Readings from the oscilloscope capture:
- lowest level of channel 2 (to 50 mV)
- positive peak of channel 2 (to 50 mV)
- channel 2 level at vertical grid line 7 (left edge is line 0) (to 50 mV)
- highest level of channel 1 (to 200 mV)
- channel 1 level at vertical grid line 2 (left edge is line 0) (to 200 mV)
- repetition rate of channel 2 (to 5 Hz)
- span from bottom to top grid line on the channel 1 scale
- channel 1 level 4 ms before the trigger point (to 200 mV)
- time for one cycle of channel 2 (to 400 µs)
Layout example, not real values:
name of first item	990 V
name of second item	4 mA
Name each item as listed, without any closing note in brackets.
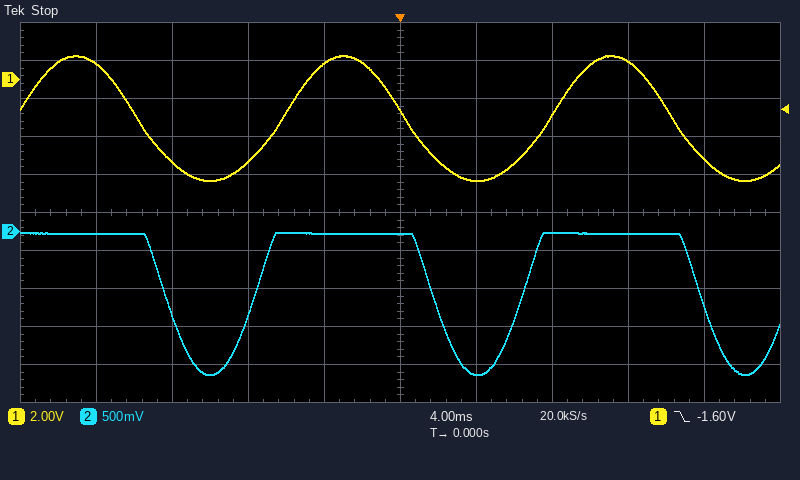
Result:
lowest level of channel 2	-1.90 V
positive peak of channel 2	0 mV
channel 2 level at vertical grid line 7 (left edge is line 0)	0 mV
highest level of channel 1	1.2 V
channel 1 level at vertical grid line 2 (left edge is line 0)	-4.4 V
repetition rate of channel 2	70 Hz
span from bottom to top grid line on the channel 1 scale	20 V
channel 1 level 4 ms before the trigger point	800 mV
time for one cycle of channel 2	14.0 ms
